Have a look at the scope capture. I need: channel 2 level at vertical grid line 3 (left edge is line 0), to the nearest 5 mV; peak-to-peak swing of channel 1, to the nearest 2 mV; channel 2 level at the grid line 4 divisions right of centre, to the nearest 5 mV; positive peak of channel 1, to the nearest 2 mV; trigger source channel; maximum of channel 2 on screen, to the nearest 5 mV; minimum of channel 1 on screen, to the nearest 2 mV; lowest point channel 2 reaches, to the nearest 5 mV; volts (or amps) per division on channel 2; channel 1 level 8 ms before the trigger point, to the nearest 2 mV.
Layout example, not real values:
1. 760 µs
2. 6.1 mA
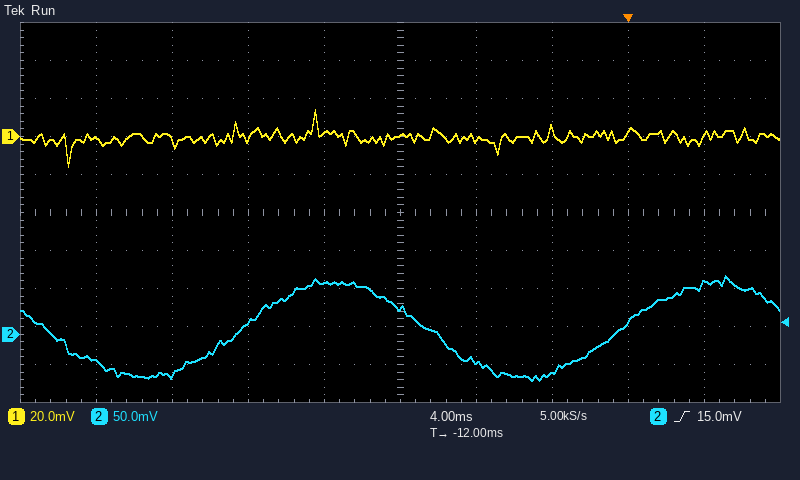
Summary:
1. 15 mV
2. 30 mV
3. 65 mV
4. 14 mV
5. channel 2
6. 75 mV
7. -16 mV
8. -60 mV
9. 50 mV
10. -2 mV
